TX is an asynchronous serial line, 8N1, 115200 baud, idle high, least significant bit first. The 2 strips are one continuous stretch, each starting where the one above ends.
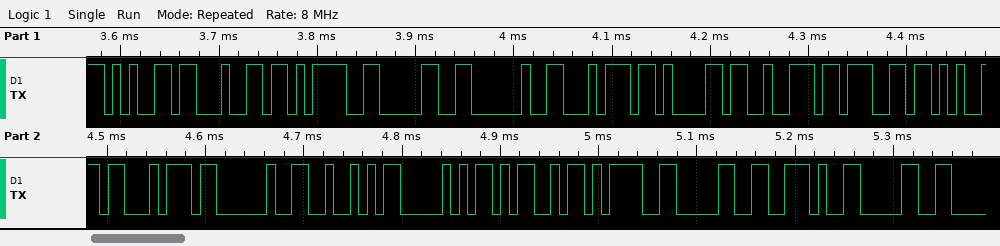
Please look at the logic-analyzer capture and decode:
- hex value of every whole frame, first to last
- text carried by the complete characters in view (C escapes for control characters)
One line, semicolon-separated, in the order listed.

65 64 3D 30 20 74 61 72 67 65 74 20 52 50 4D 3D 30 2E 30; "ed=0 target RPM=0.0"
